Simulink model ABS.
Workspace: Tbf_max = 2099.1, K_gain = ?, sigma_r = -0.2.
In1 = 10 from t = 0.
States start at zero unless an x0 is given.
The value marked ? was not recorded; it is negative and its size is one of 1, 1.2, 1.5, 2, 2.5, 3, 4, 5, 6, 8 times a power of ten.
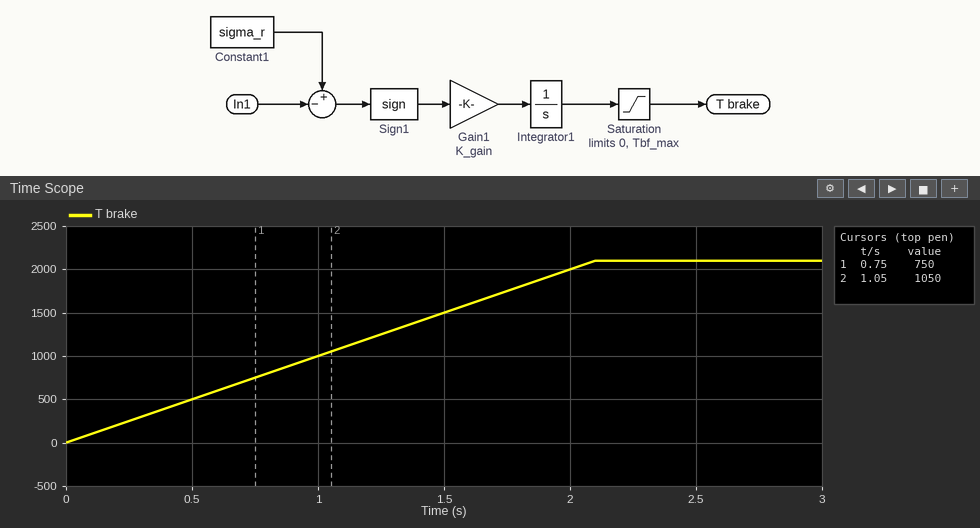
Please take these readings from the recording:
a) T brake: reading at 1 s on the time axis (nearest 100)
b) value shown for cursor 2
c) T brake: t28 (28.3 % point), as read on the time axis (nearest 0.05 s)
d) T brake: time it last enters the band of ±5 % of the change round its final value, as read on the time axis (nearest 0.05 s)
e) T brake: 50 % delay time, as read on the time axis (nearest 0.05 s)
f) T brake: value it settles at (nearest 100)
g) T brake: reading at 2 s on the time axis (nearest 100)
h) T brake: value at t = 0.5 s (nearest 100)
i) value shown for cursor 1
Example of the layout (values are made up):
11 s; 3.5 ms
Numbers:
1000; 1050; 0.60 s; 2.00 s; 1.05 s; 2100; 2000; 500; 750
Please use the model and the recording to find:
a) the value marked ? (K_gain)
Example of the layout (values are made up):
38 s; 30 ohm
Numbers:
-1000
